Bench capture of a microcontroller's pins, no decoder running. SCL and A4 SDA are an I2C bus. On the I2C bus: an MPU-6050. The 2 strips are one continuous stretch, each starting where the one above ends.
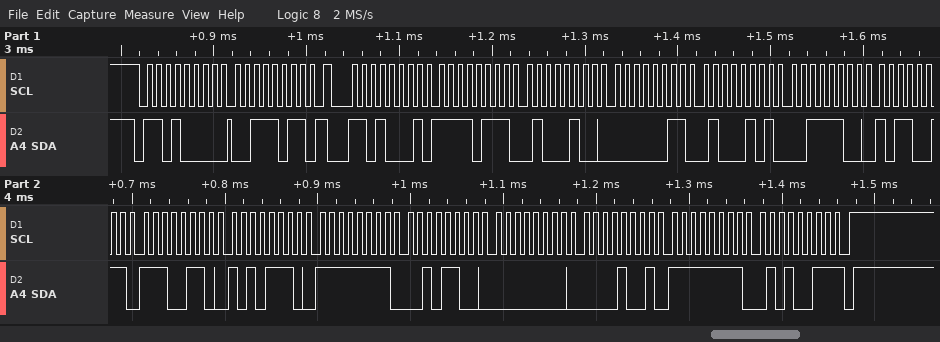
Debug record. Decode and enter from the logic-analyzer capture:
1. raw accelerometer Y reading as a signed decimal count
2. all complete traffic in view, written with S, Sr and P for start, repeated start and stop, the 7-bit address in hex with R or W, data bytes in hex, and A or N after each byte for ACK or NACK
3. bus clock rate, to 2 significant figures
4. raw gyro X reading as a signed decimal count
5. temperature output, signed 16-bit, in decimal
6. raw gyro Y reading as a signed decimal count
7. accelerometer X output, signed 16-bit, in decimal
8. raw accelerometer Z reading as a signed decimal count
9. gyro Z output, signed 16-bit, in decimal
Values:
837
S 68W A 3B A Sr 68R A F7 A 44 A 03 A 45 A 3C A B3 A E6 A AE A FF A 2C A 00 A 09 A FF A 53 N P
100 kHz
-212
-6482
9
-2236
15539
-173
